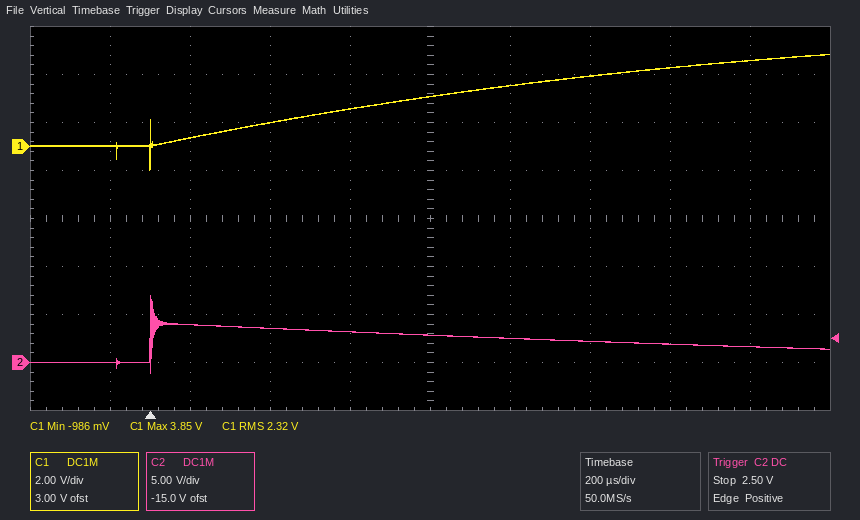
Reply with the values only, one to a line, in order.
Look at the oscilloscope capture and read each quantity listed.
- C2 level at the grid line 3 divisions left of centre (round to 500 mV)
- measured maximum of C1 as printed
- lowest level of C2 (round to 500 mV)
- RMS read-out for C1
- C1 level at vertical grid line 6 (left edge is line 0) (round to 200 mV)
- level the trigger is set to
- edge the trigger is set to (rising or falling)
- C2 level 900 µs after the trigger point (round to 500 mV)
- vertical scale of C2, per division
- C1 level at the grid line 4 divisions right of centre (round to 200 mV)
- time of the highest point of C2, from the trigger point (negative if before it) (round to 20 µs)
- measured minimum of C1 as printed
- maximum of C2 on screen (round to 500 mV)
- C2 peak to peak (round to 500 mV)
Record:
4.0 V
3.85 V
-1.0 V
2.32 V
2.6 V
2.50 V
rising
2.5 V
5 V
3.6 V
0 µs
-986 mV
7.0 V
8.0 V
